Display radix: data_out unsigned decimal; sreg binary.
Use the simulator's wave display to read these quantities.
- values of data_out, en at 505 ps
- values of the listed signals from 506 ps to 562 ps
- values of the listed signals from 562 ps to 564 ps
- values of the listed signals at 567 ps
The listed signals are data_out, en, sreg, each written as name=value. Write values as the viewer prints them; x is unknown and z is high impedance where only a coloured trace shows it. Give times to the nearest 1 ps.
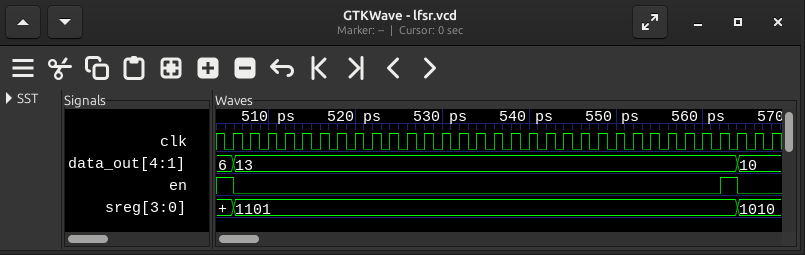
data_out=6, en=1
data_out=13, en=0, sreg=1101
data_out=13, en=1, sreg=1101
data_out=10, en=0, sreg=1010
